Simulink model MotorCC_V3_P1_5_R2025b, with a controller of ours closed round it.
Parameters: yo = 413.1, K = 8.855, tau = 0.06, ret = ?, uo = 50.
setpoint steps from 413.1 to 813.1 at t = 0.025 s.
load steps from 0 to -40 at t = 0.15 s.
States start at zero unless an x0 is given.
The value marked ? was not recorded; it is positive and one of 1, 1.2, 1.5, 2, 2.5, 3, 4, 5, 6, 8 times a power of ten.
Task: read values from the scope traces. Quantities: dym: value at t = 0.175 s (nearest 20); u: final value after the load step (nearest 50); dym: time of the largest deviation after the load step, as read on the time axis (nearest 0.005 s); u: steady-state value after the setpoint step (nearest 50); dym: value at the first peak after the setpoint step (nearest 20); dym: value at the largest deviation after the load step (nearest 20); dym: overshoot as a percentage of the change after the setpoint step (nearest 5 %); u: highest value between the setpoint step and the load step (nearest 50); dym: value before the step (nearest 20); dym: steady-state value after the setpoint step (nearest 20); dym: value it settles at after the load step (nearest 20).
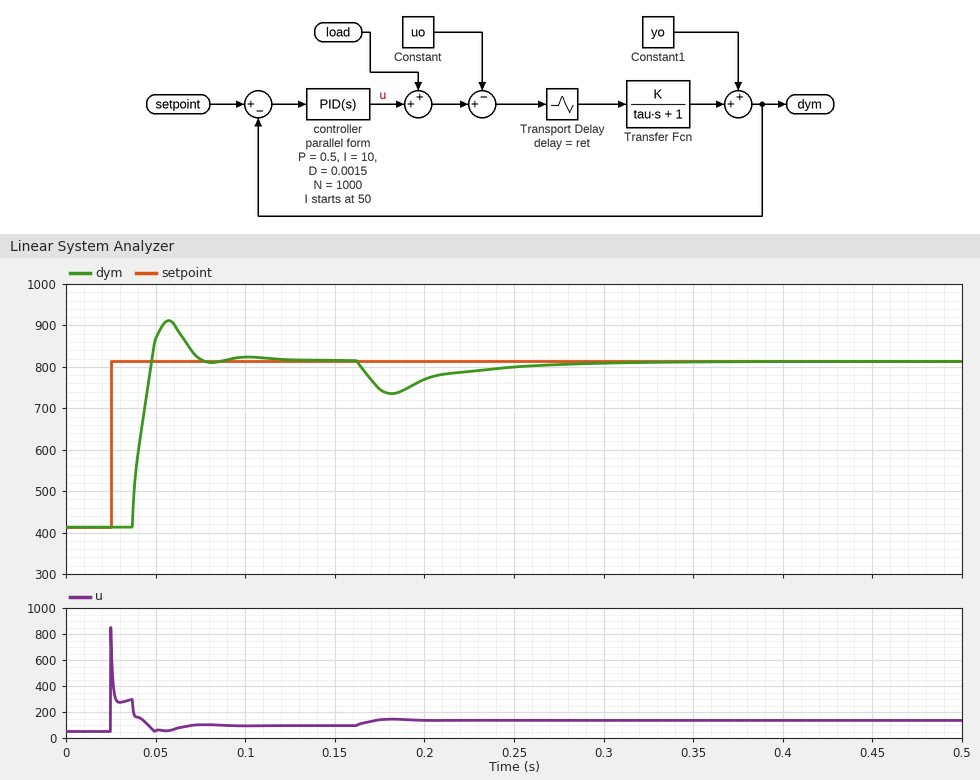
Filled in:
740
150
0.180 s
100
920
740
25 %
850
420
820
820
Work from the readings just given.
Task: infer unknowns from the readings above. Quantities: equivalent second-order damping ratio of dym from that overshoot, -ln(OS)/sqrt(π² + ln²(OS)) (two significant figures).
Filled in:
0.40
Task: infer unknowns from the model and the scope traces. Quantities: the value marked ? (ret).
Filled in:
0.012
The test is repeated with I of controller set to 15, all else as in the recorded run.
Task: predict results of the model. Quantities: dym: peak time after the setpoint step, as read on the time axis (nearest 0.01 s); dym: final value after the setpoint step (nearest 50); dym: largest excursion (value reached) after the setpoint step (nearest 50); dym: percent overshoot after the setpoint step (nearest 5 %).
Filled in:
0.06 s
800
950
35 %
